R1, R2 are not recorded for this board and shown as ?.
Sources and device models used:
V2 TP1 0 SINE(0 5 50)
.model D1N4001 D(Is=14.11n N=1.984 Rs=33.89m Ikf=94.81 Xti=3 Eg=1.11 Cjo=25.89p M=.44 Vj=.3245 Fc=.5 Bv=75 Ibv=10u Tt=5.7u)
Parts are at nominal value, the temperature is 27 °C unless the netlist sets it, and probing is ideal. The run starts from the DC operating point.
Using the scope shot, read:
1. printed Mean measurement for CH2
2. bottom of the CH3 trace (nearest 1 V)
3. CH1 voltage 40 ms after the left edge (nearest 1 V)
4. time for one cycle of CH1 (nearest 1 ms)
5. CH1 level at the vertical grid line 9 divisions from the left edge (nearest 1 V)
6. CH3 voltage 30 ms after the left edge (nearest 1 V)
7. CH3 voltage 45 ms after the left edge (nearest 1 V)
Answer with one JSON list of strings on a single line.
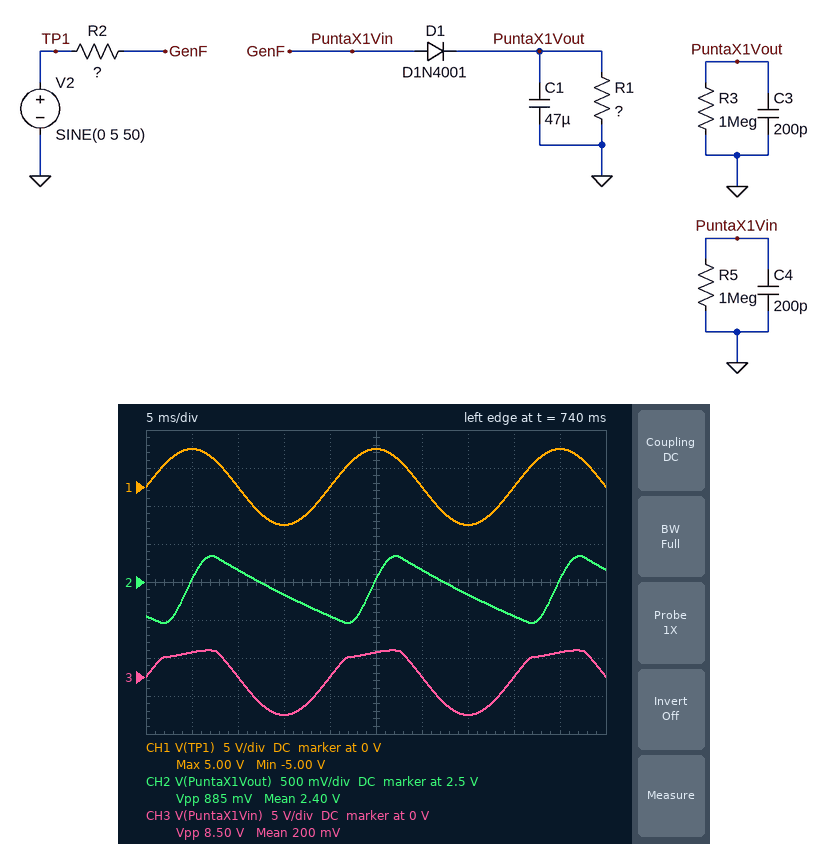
["2.40 V", "-5 V", "0 V", "20 ms", "5 V", "0 V", "3 V"]
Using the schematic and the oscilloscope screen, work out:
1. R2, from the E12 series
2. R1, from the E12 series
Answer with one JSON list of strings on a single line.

["120 Ω", "820 Ω"]
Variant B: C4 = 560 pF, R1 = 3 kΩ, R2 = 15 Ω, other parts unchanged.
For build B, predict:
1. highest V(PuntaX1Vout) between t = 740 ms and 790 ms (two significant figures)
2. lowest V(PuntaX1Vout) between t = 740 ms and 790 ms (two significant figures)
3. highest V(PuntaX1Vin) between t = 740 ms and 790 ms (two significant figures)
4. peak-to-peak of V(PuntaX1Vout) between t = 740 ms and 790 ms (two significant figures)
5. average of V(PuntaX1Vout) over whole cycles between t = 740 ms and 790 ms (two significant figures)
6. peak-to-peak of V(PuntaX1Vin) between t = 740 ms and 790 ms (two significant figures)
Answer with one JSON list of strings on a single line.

["4.2 V", "3.7 V", "4.9 V", "490 mV", "4.0 V", "9.9 V"]
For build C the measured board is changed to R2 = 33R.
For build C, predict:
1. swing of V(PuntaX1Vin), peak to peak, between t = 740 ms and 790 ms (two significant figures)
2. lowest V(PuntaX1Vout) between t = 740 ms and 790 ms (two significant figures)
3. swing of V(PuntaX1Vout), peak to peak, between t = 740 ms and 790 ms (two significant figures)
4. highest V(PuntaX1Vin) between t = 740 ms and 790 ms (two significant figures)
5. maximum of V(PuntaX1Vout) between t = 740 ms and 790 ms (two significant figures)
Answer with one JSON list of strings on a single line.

["9.5 V", "2.5 V", "1.3 V", "4.5 V", "3.8 V"]
